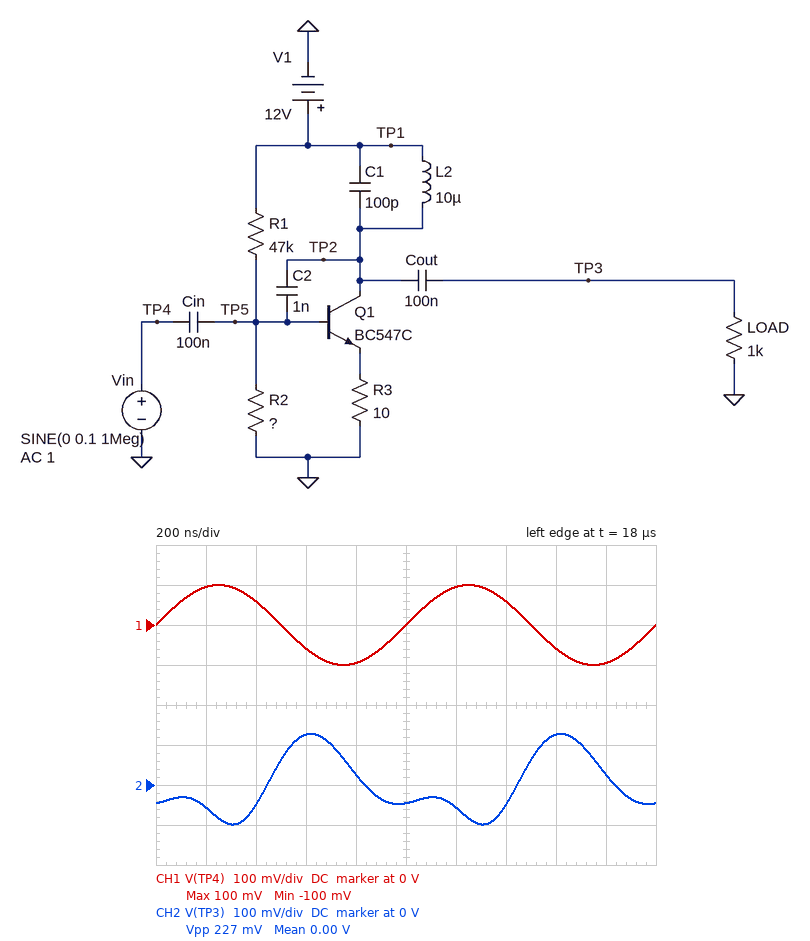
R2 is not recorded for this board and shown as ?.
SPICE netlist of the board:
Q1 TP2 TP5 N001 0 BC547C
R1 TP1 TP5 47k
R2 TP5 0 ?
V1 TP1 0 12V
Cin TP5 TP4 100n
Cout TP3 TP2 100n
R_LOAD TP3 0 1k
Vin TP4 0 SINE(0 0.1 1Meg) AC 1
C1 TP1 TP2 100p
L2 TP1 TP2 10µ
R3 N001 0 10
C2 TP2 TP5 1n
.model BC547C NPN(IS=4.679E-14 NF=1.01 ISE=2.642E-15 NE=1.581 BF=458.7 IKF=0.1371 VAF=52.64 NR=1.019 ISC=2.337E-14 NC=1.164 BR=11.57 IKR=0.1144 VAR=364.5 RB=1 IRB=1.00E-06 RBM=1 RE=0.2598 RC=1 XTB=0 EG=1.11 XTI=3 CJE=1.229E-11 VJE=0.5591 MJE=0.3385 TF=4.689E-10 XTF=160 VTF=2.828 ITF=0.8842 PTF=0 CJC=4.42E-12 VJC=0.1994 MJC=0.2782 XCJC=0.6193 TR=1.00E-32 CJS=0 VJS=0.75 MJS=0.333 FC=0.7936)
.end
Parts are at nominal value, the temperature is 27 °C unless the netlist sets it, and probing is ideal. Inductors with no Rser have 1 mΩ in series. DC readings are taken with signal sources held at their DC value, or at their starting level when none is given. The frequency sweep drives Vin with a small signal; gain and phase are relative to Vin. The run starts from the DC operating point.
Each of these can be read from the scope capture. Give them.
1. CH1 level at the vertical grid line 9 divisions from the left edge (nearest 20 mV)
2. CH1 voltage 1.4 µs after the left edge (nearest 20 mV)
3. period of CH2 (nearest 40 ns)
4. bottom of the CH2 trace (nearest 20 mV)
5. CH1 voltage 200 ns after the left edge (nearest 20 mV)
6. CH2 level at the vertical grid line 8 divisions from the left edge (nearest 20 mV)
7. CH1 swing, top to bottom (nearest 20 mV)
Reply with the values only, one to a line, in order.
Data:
-100 mV
60 mV
1.00 µs
-100 mV
100 mV
120 mV
200 mV
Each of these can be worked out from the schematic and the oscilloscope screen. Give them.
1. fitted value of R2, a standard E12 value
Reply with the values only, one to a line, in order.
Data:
2.2 kΩ
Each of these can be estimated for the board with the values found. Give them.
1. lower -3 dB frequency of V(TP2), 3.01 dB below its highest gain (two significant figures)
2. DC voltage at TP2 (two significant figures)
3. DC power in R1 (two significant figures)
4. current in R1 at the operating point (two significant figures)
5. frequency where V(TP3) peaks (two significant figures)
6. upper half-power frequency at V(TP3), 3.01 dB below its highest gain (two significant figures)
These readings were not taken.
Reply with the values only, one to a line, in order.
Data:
1.5 MHz
12 V
2.8 mW
240 µA
1.5 MHz
1.6 MHz
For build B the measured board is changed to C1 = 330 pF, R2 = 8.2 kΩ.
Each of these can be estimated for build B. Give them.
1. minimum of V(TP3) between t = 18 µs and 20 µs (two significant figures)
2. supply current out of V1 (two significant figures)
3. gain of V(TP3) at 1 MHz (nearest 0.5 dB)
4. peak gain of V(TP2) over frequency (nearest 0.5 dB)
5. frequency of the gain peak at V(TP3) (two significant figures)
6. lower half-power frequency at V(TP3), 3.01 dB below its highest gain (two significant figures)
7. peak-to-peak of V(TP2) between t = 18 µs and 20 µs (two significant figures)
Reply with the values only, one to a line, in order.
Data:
-1.1 V
41 mA
21.0 dB
33.5 dB
1.4 MHz
1.3 MHz
2.3 V
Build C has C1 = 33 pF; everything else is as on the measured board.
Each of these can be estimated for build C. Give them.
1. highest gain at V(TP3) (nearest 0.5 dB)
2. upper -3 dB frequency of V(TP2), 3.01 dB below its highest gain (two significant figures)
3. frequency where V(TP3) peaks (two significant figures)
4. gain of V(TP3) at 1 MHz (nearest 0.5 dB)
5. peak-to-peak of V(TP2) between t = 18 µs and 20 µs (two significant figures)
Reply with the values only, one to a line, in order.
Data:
20.0 dB
1.7 MHz
1.6 MHz
-3.5 dB
240 mV
